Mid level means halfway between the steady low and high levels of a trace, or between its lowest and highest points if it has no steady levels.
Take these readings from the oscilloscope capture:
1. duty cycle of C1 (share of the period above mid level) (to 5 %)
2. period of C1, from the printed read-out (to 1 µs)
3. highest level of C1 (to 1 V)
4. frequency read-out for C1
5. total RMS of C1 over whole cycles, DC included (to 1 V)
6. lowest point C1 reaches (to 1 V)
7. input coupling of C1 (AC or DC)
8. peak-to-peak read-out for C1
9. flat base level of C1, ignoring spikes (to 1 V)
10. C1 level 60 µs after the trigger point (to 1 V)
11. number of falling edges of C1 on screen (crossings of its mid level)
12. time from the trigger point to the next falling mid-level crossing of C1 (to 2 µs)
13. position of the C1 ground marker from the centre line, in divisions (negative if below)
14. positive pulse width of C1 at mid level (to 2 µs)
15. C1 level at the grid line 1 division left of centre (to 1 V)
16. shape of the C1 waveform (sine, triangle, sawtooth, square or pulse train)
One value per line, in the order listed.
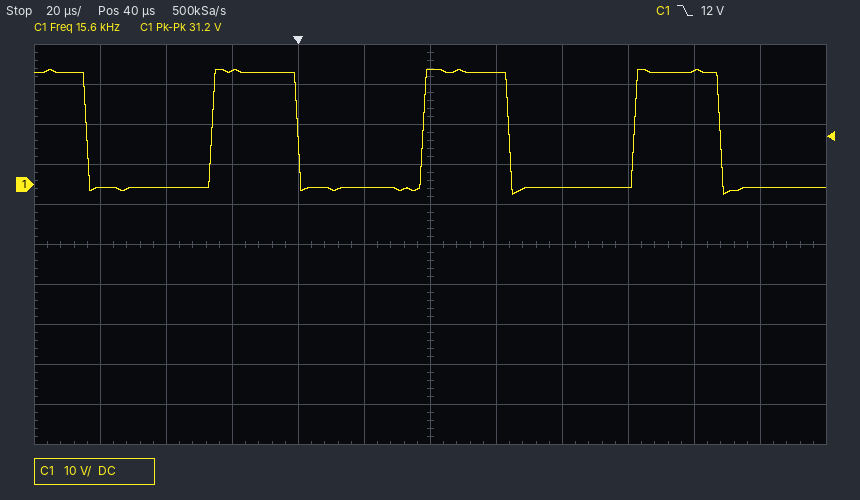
40 %
64 µs
29 V
15.6 kHz
18 V
-2 V
DC
31.2 V
-1 V
28 V
4
64 µs
+1.5 div
26 µs
-1 V
pulse train
